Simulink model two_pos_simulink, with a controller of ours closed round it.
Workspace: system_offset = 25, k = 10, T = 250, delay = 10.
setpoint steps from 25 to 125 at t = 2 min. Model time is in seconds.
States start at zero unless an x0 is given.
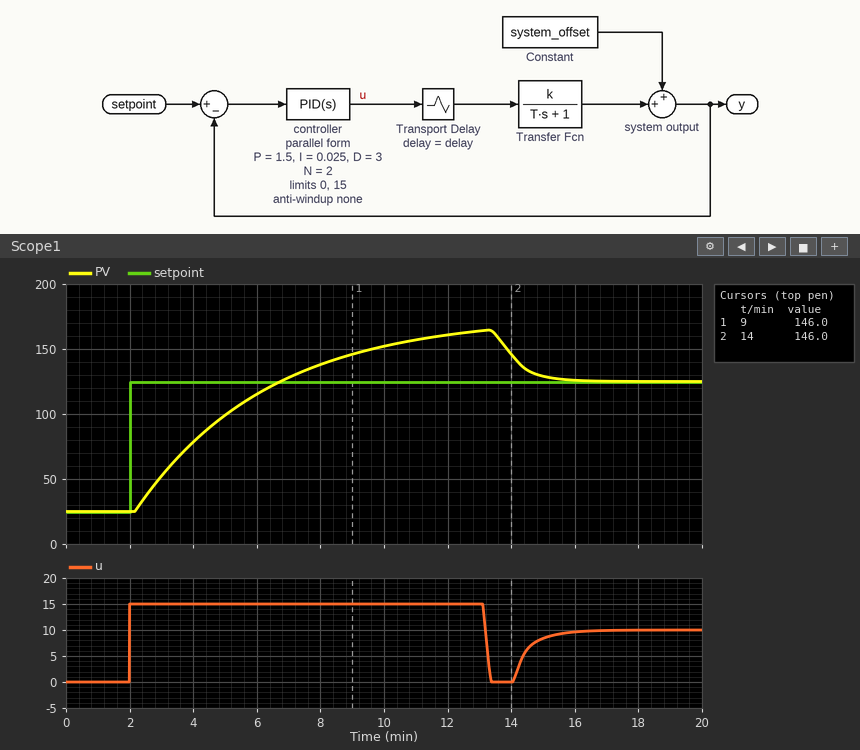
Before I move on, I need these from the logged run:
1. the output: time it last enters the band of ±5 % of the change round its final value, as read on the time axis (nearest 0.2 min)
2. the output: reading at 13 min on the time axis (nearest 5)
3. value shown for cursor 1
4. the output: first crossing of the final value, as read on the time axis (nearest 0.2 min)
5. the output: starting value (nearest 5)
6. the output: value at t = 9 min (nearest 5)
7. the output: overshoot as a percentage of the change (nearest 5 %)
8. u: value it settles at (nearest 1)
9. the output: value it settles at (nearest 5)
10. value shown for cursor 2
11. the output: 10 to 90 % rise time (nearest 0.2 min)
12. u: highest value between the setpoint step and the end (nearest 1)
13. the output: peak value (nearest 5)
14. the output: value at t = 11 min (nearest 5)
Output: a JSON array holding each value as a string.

["14.8 min", "165", "146.0", "6.8 min", "25", "145", "40 %", "10", "125", "146.0", "3.6 min", "15", "165", "155"]
